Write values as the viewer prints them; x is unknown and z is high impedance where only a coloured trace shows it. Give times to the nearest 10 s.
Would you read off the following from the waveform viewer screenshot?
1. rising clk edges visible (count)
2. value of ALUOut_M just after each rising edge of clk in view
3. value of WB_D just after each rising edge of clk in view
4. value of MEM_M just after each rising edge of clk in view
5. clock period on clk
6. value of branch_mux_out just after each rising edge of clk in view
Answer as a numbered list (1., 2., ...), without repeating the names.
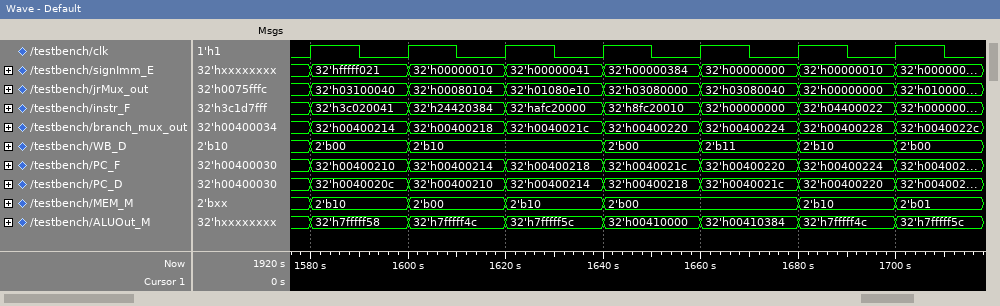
1. 7
2. 32'h7fffff58, 32'h7fffff4c, 32'h7fffff5c, 32'h00410000, 32'h00410384, 32'h7fffff4c, 32'h7fffff5c
3. 2'b00, 2'b10, 2'b10, 2'b00, 2'b11, 2'b10, 2'b00
4. 2'b10, 2'b00, 2'b10, 2'b00, 2'b00, 2'b10, 2'b01
5. 20 s
6. 32'h00400214, 32'h00400218, 32'h0040021c, 32'h00400220, 32'h00400224, 32'h00400228, 32'h0040022c
